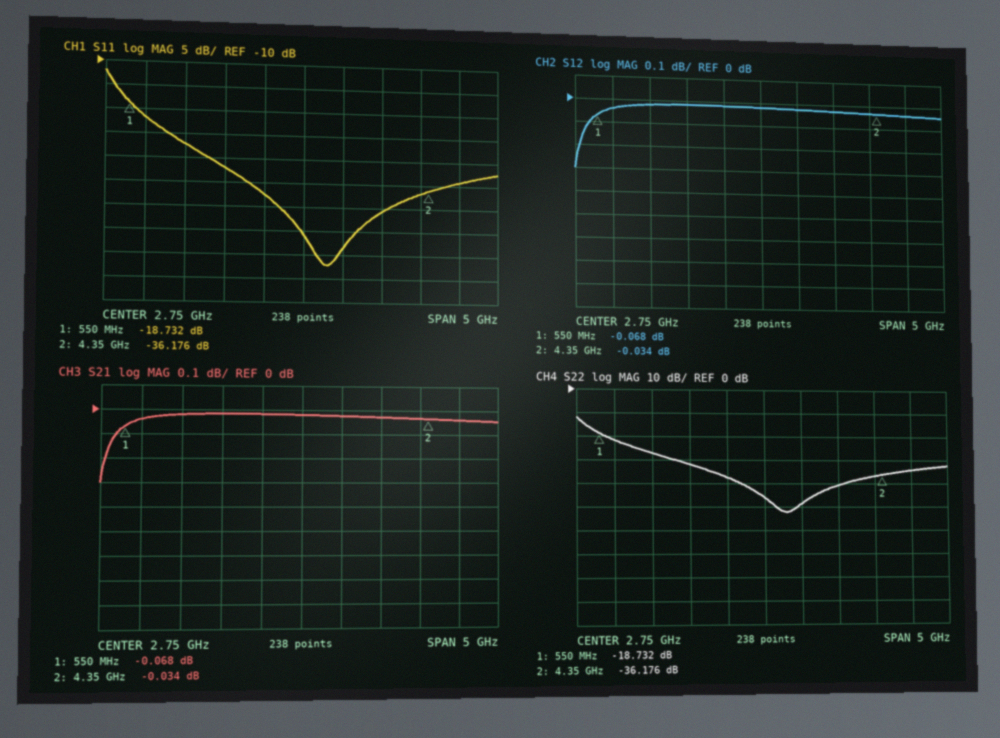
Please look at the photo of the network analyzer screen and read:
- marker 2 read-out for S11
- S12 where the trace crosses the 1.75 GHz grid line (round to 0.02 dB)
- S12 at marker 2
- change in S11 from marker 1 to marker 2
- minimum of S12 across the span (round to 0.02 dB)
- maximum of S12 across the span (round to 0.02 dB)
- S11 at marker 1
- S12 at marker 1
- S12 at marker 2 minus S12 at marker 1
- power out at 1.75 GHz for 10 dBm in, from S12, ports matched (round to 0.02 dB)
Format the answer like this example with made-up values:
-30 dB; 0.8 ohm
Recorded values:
-36.176 dB; -0.02 dB; -0.034 dB; -17.444 dB; -0.30 dB; -0.02 dB; -18.732 dB; -0.068 dB; 0.034 dB; 9.98 dBm
